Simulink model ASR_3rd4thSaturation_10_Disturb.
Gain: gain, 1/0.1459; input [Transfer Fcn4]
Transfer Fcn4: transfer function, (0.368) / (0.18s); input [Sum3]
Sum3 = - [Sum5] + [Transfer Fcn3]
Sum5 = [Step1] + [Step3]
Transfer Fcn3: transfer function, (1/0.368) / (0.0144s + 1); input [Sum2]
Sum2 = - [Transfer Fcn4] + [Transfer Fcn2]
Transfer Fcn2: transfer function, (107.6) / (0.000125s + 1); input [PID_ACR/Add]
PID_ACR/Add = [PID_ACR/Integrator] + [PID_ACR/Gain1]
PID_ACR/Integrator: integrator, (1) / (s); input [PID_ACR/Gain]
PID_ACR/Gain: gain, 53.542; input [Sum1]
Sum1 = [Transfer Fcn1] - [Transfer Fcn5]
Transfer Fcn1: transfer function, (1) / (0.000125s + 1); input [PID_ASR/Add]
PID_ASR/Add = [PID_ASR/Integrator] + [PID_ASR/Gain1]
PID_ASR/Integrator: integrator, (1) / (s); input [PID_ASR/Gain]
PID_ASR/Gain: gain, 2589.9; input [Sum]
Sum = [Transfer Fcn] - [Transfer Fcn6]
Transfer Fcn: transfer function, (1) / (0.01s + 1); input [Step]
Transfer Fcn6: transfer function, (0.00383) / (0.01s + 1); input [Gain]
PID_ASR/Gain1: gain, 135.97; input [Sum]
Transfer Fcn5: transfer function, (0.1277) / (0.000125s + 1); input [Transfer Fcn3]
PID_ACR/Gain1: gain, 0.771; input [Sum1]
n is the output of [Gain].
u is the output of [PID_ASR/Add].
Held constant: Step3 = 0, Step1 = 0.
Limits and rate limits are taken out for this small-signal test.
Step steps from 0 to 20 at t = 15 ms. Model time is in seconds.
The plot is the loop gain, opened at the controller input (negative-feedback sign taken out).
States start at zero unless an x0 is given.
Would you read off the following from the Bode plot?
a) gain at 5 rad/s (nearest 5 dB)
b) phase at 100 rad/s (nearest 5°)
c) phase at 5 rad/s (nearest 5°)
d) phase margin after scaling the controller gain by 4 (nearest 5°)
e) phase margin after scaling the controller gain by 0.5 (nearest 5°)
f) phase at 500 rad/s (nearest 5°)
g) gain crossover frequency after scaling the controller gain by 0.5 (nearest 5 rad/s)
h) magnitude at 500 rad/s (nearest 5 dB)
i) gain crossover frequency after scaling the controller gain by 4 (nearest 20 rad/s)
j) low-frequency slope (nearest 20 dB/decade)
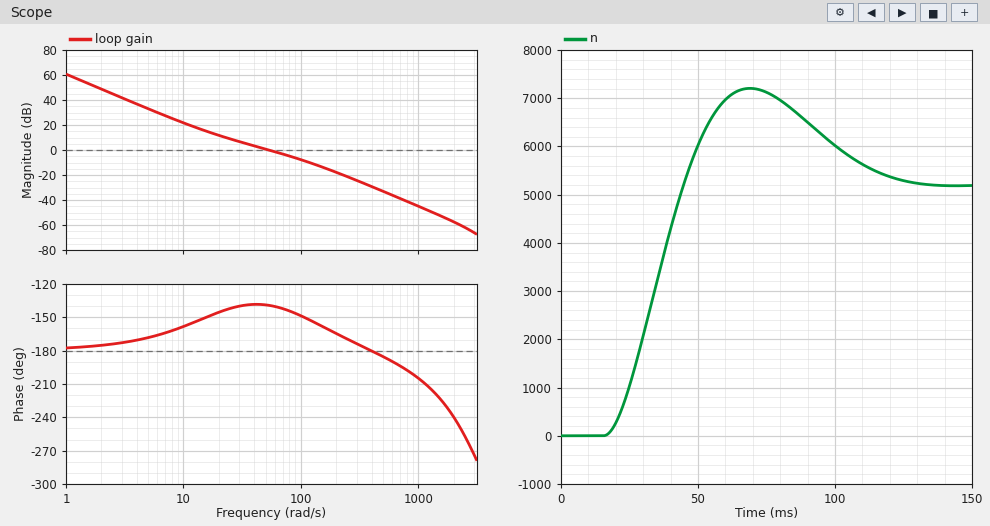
35 dB
-150°
-170°
25°
40°
-185°
30 rad/s
-35 dB
140 rad/s
-40 dB/decade
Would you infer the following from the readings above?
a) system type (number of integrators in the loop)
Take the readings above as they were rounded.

2
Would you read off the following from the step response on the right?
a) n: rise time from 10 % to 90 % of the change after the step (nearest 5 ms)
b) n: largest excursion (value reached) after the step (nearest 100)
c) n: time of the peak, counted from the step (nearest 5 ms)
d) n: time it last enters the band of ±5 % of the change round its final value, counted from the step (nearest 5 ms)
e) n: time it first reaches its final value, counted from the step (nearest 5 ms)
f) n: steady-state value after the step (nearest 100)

20 ms
7200
55 ms
100 ms
30 ms
5200
